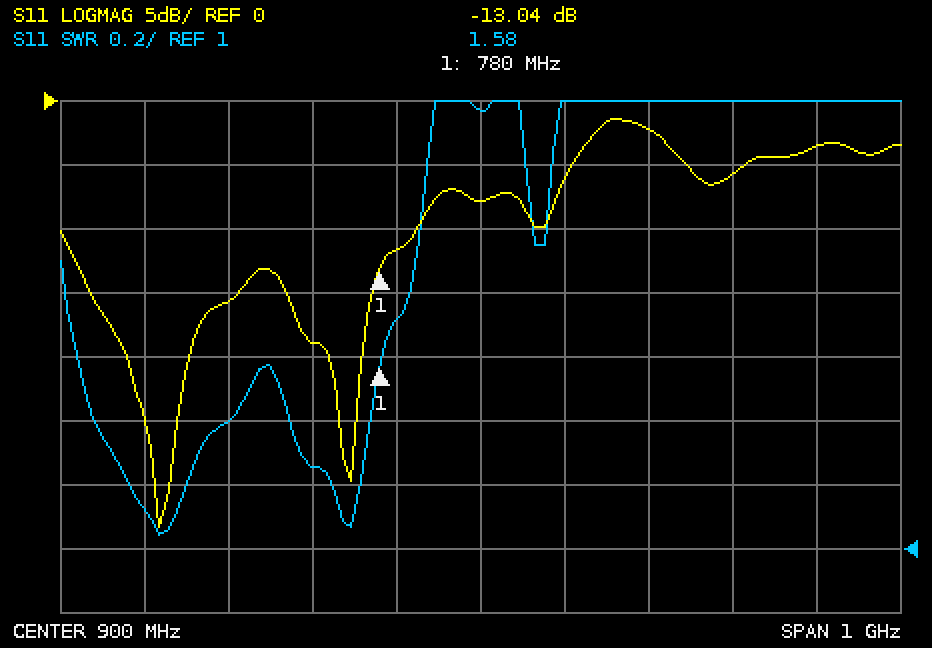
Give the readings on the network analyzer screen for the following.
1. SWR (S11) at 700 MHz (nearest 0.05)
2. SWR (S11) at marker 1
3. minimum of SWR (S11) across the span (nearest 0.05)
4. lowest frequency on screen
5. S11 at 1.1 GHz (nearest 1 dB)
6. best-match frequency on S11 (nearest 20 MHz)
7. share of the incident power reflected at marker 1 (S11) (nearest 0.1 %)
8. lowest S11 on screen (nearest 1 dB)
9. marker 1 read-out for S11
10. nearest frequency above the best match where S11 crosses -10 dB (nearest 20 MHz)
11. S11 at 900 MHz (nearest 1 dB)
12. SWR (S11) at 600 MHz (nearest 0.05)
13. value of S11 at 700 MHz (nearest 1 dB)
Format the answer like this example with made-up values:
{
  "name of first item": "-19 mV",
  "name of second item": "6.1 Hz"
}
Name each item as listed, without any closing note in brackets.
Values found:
{
  "SWR (S11) at 700 MHz": "1.25",
  "SWR (S11) at marker 1": "1.58",
  "minimum of SWR (S11) across the span": "1.05",
  "lowest frequency on screen": "400 MHz",
  "S11 at 1.1 GHz": "-2 dB",
  "best-match frequency on S11": "520 MHz",
  "share of the incident power reflected at marker 1 (S11)": "5.0 %",
  "lowest S11 on screen": "-33 dB",
  "marker 1 read-out for S11": "-13.04 dB",
  "nearest frequency above the best match where S11 crosses -10 dB": "820 MHz",
  "S11 at 900 MHz": "-8 dB",
  "SWR (S11) at 600 MHz": "1.40",
  "value of S11 at 700 MHz": "-19 dB"
}
